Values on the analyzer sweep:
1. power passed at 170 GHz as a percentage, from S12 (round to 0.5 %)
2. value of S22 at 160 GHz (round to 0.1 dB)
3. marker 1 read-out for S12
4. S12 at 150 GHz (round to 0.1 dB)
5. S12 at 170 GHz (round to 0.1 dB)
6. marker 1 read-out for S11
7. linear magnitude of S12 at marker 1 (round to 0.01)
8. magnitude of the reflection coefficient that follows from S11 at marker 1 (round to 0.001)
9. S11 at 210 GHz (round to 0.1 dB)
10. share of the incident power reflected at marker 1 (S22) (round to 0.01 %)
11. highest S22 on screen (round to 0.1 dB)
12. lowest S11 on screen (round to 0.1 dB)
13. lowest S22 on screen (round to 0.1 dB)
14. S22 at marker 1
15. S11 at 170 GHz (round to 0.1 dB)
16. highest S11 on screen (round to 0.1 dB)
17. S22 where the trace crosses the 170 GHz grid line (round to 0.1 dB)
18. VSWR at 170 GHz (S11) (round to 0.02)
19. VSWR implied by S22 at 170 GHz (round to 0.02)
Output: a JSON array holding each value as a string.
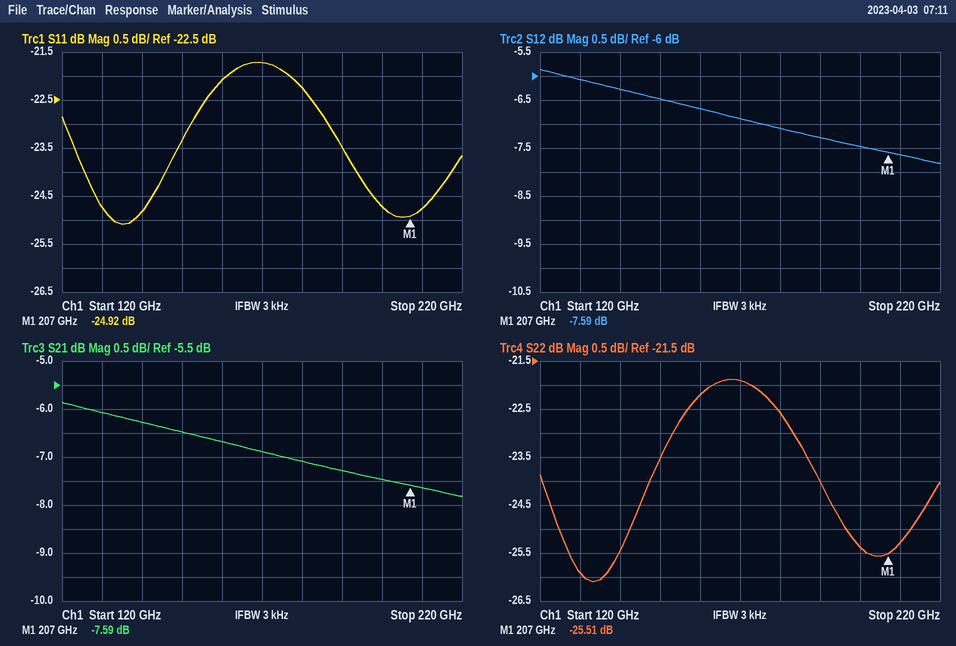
["20.5 %", "-22.2 dB", "-7.59 dB", "-6.5 dB", "-6.9 dB", "-24.92 dB", "0.42", "0.057", "-24.8 dB", "0.28 %", "-21.9 dB", "-25.1 dB", "-26.1 dB", "-25.51 dB", "-21.7 dB", "-21.7 dB", "-21.9 dB", "1.18", "1.18"]
